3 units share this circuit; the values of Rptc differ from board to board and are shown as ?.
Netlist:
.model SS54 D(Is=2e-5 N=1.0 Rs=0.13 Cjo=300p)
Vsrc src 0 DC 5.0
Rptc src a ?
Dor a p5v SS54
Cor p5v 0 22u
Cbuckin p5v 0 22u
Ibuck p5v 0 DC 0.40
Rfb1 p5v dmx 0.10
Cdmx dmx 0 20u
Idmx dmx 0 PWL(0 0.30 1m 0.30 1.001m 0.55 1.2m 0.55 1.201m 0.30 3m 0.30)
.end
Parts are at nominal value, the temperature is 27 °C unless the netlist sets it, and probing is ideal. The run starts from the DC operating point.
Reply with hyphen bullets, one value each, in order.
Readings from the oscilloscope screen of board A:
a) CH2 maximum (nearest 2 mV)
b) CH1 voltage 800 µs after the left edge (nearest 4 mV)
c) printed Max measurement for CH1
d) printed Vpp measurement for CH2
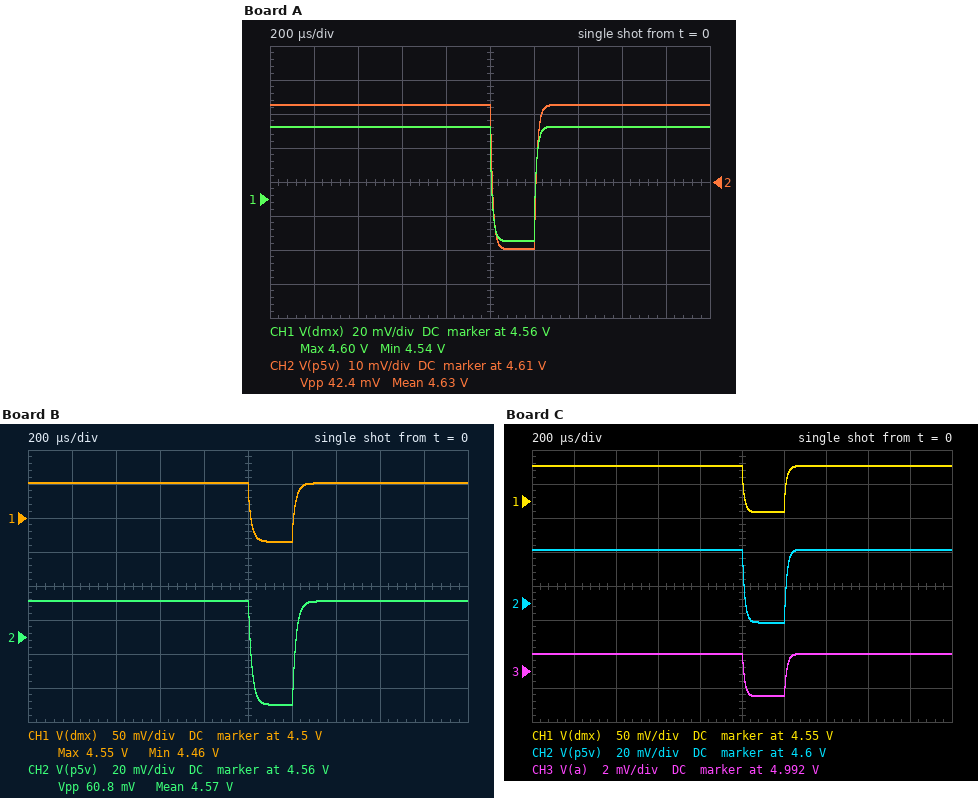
- 4.632 V
- 4.604 V
- 4.60 V
- 42.4 mV
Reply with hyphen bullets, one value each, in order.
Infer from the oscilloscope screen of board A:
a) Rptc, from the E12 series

- 8.2 mΩ
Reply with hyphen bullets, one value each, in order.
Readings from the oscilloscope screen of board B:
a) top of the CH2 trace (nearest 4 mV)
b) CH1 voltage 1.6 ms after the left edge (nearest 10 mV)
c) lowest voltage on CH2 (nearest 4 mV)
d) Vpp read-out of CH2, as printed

- 4.580 V
- 4.55 V
- 4.520 V
- 60.8 mV
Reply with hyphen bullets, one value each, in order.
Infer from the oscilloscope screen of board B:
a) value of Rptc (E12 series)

- 0.082 Ω
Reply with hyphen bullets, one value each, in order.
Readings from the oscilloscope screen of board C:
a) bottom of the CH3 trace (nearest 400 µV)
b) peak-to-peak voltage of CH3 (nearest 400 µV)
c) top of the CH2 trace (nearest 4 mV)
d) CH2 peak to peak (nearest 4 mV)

- 4.9904 V
- 2.4 mV
- 4.632 V
- 44 mV
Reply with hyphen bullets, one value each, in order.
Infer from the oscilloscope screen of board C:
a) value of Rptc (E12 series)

- 0.01 Ω
